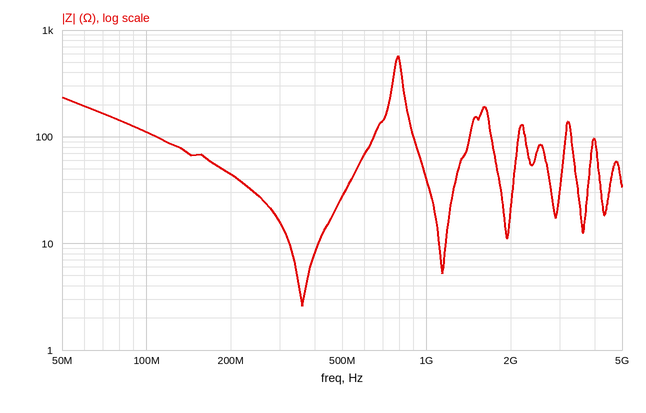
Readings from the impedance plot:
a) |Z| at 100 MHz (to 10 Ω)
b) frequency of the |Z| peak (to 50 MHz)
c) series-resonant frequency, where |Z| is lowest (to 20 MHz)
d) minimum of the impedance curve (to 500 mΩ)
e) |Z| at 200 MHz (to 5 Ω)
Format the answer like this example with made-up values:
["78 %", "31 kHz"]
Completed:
["110 Ω", "800 MHz", "360 MHz", "2.5 Ω", "45 Ω"]
